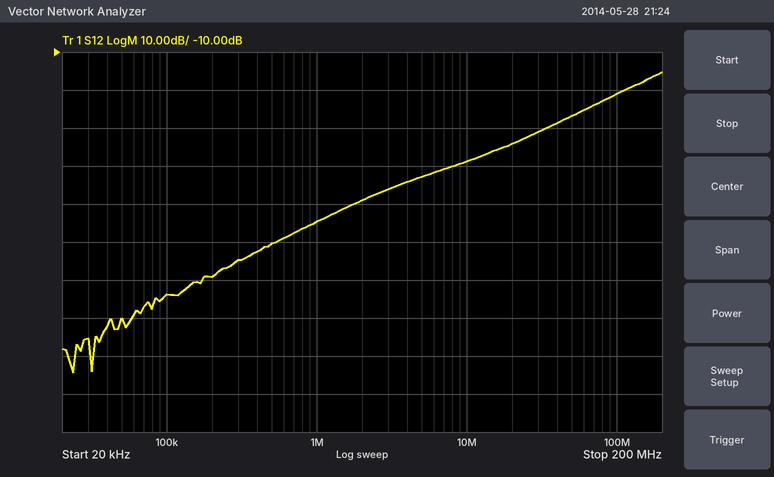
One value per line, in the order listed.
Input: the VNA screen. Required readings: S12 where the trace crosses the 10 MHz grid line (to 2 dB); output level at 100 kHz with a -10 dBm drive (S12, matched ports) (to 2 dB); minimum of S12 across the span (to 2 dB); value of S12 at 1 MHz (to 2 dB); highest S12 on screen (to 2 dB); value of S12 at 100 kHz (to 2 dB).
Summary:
-38 dB
-84 dBm
-94 dB
-54 dB
-16 dB
-74 dB
